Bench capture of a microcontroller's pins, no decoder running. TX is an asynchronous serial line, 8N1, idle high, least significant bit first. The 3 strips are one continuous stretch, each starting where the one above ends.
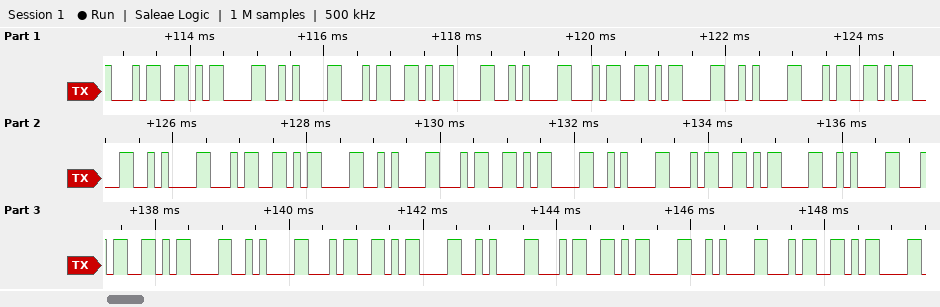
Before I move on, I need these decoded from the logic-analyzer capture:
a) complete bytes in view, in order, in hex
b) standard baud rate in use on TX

0x34 0x0D 0x0A 0x34 0x0D 0x0A 0x34 0x0D 0x0A 0x34 0x0D 0x0A 0x34 0x0D 0x0A 0x34 0x0D 0x0A 0x34 0x0D 0x0A 0x34 0x0D 0x0A 0x34 0x0D 0x0A 0x34 0x0D 0x0A 0x34 0x0D
9600 baud
